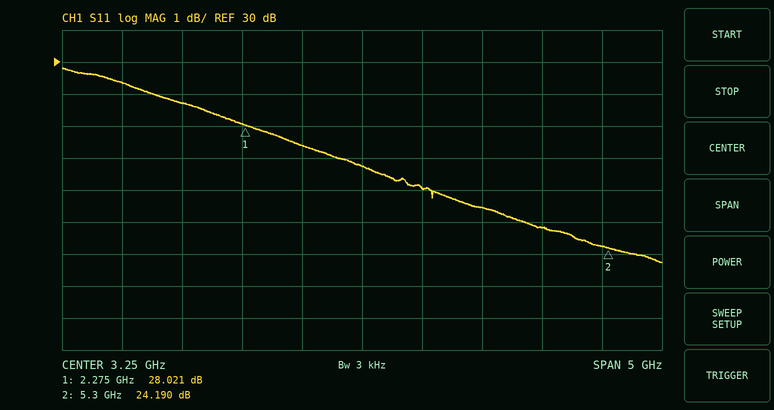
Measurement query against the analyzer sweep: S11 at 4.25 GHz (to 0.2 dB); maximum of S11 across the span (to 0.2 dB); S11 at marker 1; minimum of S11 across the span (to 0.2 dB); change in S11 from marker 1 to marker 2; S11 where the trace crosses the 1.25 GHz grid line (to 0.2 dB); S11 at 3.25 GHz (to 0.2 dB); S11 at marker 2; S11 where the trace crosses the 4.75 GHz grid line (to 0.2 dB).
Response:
25.4 dB
29.8 dB
28.021 dB
23.8 dB
-3.831 dB
29.4 dB
26.8 dB
24.190 dB
24.8 dB
